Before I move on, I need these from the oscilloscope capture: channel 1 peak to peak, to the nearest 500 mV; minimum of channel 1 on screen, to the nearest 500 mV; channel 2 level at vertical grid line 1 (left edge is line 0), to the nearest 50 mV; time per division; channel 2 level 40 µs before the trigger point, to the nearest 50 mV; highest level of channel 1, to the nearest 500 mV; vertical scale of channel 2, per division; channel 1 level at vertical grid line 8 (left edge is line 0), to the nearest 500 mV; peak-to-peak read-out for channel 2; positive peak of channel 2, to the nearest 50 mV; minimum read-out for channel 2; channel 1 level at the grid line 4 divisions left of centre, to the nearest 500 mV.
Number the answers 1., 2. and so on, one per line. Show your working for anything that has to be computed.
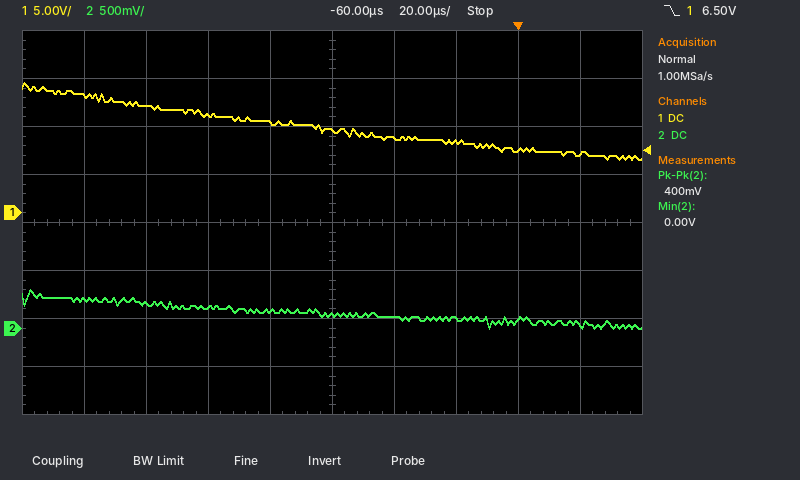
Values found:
1. 13.5 V − (5.5 V) = 8.0 V
2. 5.5 V
3. 300 mV
4. 20 µs
5. 100 mV
6. 13.5 V
7. 500 mV
8. 6.5 V
9. 400 mV
10. 400 mV
11. 0.00 V
12. 12.0 V
